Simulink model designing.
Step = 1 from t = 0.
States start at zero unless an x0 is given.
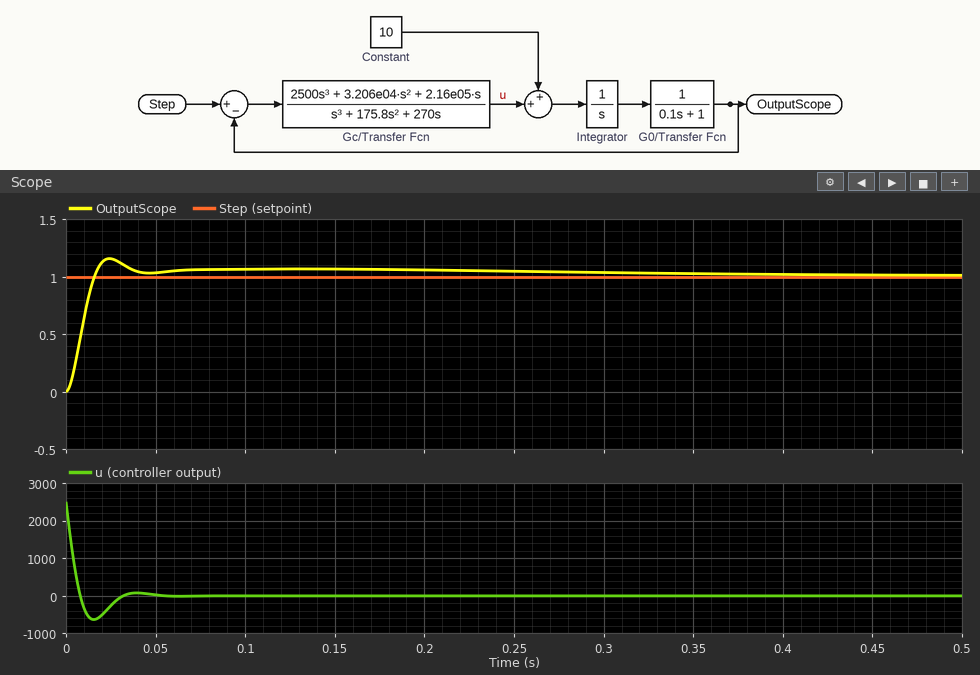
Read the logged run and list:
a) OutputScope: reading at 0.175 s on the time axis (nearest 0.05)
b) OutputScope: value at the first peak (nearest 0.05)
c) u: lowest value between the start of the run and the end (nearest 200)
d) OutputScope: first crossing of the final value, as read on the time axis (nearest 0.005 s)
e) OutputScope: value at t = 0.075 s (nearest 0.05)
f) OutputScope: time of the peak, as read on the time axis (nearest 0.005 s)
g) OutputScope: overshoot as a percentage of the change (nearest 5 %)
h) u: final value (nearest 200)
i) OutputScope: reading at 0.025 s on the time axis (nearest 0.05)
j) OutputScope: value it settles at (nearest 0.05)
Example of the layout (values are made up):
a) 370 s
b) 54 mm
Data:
a) 1.05
b) 1.15
c) -600
d) 0.015 s
e) 1.05
f) 0.025 s
g) 15 %
h) 0
i) 1.15
j) 1.00
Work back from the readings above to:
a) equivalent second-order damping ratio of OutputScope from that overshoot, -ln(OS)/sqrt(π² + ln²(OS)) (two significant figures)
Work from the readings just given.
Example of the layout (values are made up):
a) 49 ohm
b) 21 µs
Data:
a) 0.52
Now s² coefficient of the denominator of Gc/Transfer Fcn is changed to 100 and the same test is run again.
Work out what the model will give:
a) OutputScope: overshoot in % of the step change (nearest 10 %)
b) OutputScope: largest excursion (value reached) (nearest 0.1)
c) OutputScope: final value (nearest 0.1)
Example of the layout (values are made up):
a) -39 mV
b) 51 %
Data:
a) 40 %
b) 1.4
c) 1.0
